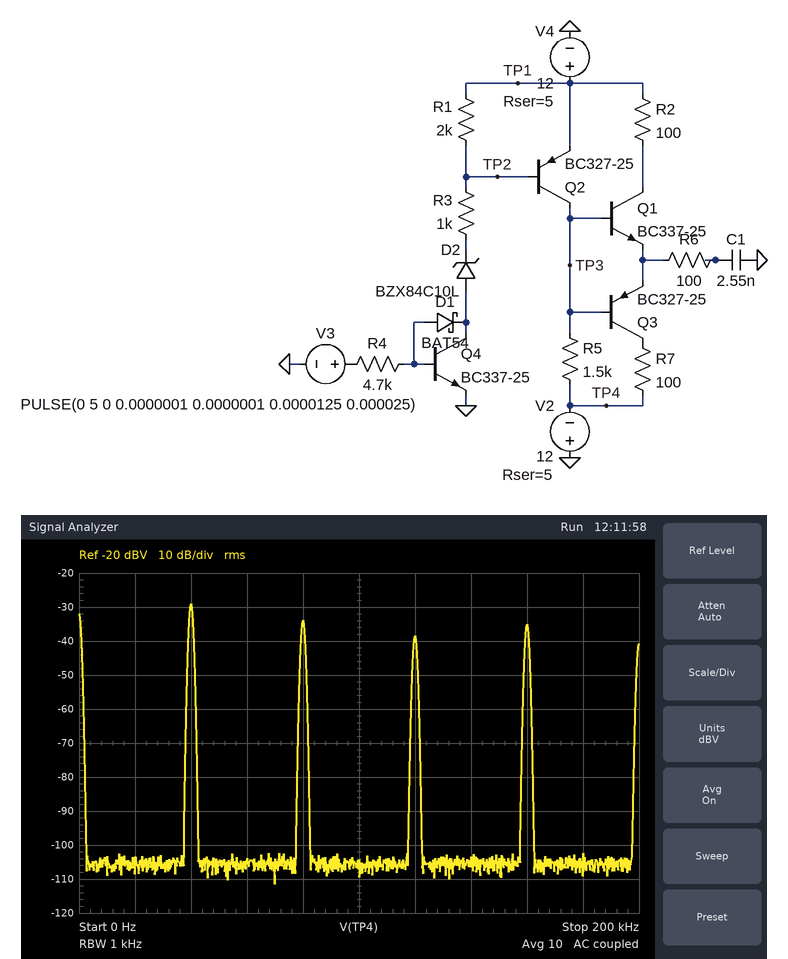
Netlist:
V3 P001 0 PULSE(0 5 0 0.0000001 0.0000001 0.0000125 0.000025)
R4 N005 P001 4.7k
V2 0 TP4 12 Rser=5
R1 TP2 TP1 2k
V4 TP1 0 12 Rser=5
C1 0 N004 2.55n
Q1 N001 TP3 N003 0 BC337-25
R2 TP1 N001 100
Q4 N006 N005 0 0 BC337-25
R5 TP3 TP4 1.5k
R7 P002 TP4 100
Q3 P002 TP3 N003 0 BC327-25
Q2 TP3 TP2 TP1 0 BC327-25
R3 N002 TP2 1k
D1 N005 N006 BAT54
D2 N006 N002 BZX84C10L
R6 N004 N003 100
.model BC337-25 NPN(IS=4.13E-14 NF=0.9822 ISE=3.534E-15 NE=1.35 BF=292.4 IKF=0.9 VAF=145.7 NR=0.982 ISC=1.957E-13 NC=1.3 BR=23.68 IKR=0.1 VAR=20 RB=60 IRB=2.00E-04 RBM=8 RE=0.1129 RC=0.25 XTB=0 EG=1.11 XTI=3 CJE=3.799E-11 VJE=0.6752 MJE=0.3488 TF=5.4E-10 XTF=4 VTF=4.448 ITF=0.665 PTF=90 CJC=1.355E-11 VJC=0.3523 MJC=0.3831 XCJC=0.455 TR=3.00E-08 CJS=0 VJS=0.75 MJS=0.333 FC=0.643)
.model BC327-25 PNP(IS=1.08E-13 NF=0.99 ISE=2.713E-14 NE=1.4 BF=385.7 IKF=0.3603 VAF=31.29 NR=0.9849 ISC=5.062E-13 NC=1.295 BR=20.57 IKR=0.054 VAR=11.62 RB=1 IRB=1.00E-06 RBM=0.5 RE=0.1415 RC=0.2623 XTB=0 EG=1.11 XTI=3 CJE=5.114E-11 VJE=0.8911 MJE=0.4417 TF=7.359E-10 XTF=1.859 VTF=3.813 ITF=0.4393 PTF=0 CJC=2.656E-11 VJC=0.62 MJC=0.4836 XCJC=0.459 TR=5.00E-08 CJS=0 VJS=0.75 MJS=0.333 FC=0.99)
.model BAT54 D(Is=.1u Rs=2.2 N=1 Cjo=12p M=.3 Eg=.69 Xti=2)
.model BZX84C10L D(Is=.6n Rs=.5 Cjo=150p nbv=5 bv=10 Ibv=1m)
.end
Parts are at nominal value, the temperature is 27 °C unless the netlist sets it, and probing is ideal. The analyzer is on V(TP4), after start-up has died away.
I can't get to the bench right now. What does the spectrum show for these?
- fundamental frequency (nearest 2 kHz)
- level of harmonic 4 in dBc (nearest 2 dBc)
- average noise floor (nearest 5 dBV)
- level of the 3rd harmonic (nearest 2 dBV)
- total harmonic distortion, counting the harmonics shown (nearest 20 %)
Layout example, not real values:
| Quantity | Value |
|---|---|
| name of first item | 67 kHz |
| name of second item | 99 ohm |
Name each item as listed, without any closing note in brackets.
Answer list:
| Quantity | Value |
|---|---|
| fundamental frequency | 40 kHz |
| level of harmonic 4 in dBc | -6 dBc |
| average noise floor | -105 dBV |
| level of the 3rd harmonic | -38 dBV |
| total harmonic distortion, counting the harmonics shown | 80 % |
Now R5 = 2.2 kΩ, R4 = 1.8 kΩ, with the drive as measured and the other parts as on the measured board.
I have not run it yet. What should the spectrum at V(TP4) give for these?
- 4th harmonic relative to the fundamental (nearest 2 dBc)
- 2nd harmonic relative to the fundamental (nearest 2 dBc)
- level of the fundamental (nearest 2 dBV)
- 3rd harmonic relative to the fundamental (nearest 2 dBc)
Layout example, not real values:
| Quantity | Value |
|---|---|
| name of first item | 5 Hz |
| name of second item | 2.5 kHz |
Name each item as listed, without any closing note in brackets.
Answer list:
| Quantity | Value |
|---|---|
| 4th harmonic relative to the fundamental | -4 dBc |
| 2nd harmonic relative to the fundamental | -2 dBc |
| level of the fundamental | -32 dBV |
| 3rd harmonic relative to the fundamental | -6 dBc |
